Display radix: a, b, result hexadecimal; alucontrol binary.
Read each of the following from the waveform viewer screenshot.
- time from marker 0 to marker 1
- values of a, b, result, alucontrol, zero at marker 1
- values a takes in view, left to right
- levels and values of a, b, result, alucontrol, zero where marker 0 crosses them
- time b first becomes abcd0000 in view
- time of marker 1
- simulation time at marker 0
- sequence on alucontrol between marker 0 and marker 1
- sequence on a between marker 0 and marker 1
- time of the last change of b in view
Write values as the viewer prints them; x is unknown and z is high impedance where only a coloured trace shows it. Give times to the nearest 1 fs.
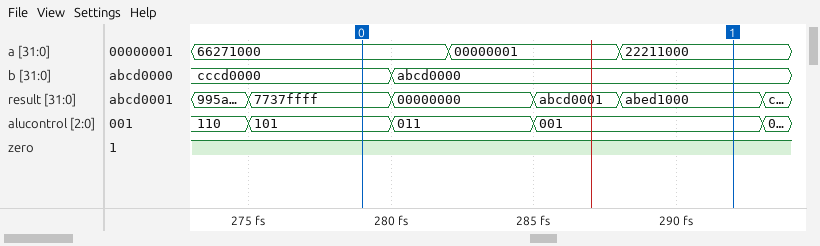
13 fs
a=22211000, b=abcd0000, result=abed1000, alucontrol=001, zero=1
66271000, 00000001, 22211000
a=66271000, b=cccd0000, result=7737ffff, alucontrol=101, zero=1
280 fs
292 fs
279 fs
101, 011, 001
66271000, 00000001, 22211000
280 fs
